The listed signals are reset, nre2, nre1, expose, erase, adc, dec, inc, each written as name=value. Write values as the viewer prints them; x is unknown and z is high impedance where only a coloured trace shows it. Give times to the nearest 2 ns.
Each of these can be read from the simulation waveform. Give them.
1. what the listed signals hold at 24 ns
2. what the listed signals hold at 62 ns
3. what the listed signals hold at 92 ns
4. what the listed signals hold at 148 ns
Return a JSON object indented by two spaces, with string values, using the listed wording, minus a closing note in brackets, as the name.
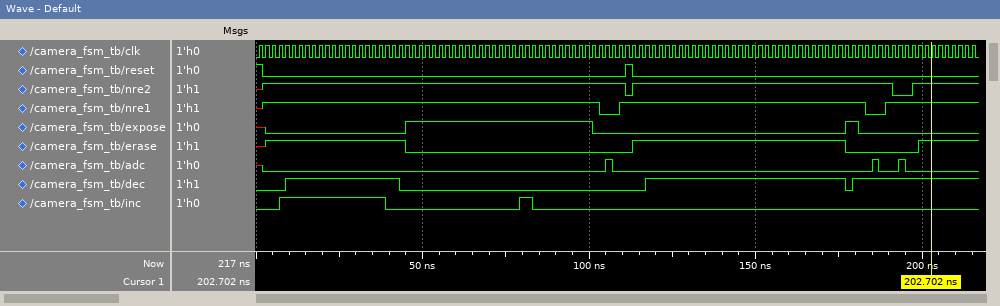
{
  "what the listed signals hold at 24 ns": "reset=0, nre2=1, nre1=1, expose=0, erase=1, adc=0, dec=1, inc=1",
  "what the listed signals hold at 62 ns": "reset=0, nre2=1, nre1=1, expose=1, erase=0, adc=0, dec=0, inc=0",
  "what the listed signals hold at 92 ns": "reset=0, nre2=1, nre1=1, expose=1, erase=0, adc=0, dec=0, inc=0",
  "what the listed signals hold at 148 ns": "reset=0, nre2=1, nre1=1, expose=0, erase=1, adc=0, dec=1, inc=0"
}
